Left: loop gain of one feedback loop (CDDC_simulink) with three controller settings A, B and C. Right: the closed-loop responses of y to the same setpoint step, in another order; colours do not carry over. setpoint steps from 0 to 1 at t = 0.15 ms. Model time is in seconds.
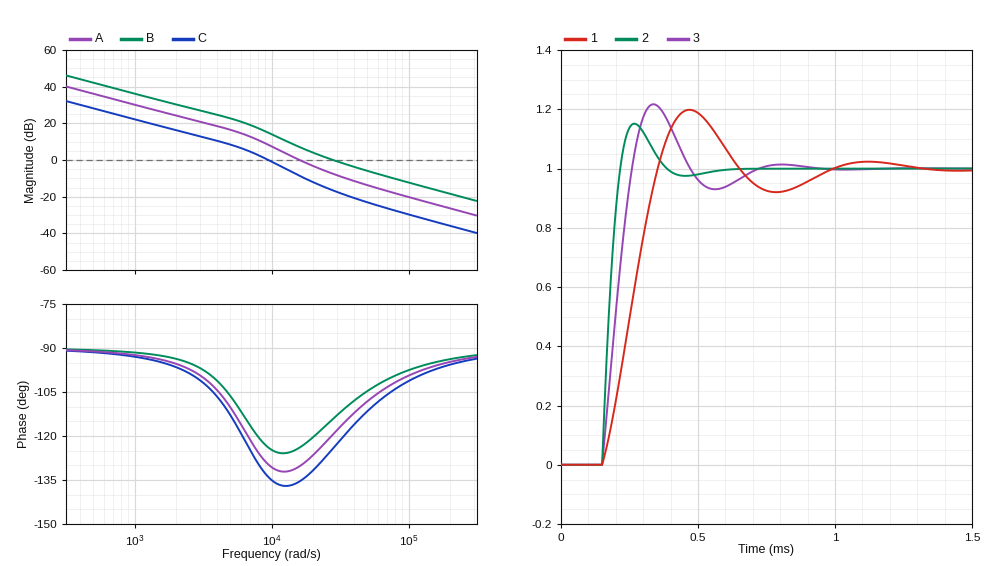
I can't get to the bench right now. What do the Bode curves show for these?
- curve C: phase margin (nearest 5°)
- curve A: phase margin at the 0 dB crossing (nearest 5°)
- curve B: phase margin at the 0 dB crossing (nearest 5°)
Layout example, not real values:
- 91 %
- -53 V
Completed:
- 45°
- 50°
- 65°
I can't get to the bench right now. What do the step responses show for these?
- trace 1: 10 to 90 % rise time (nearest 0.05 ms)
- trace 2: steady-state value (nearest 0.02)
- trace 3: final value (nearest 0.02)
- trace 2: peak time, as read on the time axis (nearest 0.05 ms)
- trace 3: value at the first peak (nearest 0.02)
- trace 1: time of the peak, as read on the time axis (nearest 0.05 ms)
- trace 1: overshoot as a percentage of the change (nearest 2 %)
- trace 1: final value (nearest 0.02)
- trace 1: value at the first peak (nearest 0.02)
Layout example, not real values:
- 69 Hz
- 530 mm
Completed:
- 0.15 ms
- 1.00
- 1.00
- 0.25 ms
- 1.22
- 0.45 ms
- 20 %
- 1.00
- 1.20
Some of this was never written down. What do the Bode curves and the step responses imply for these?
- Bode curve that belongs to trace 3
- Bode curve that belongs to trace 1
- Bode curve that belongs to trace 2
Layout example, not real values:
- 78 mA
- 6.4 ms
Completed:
- A
- C
- B
